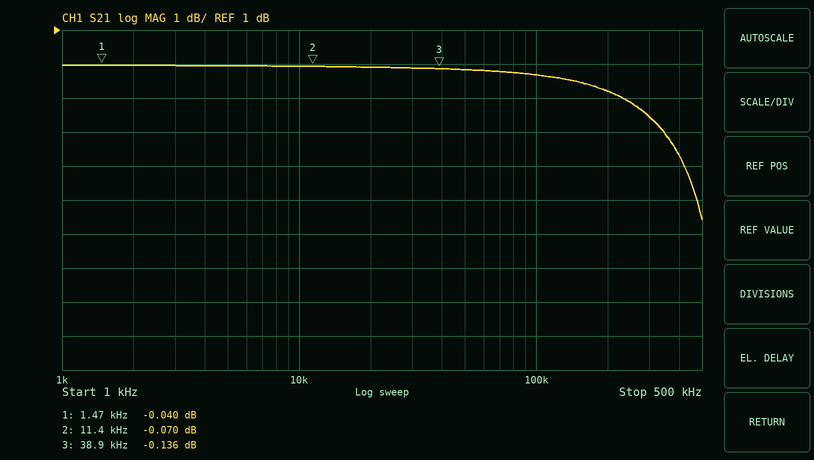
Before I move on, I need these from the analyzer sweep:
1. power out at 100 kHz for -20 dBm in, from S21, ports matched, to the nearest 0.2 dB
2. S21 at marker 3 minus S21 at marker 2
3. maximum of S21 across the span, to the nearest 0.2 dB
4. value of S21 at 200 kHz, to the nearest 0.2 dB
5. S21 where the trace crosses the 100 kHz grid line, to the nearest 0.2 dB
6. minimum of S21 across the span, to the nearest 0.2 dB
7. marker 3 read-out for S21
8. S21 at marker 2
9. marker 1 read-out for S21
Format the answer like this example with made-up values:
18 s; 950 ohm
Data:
-20.4 dBm; -0.066 dB; 0.0 dB; -0.8 dB; -0.4 dB; -4.6 dB; -0.136 dB; -0.070 dB; -0.040 dB
